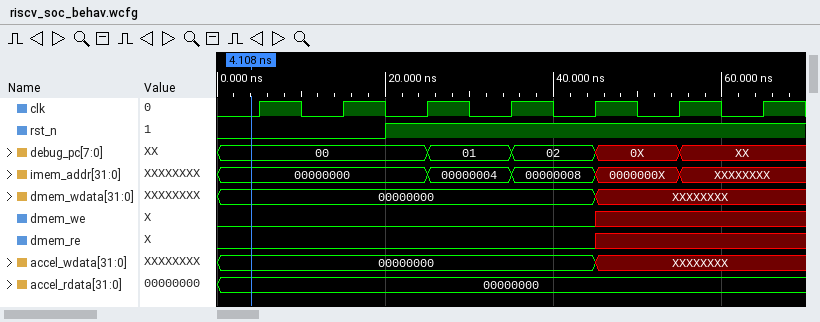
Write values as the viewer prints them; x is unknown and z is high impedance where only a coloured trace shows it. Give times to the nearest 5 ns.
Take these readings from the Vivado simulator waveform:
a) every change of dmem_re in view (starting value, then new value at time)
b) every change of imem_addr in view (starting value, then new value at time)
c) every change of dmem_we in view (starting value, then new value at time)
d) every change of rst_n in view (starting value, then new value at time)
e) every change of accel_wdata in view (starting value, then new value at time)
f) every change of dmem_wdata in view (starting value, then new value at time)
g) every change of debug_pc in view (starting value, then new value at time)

0, x at 45 ns
00000000, 00000004 at 25 ns, 00000008 at 35 ns, 0000000X at 45 ns, XXXXXXXX at 55 ns
0, x at 45 ns
0, 1 at 20 ns
00000000, XXXXXXXX at 45 ns
00000000, XXXXXXXX at 45 ns
00, 01 at 25 ns, 02 at 35 ns, 0X at 45 ns, XX at 55 ns
